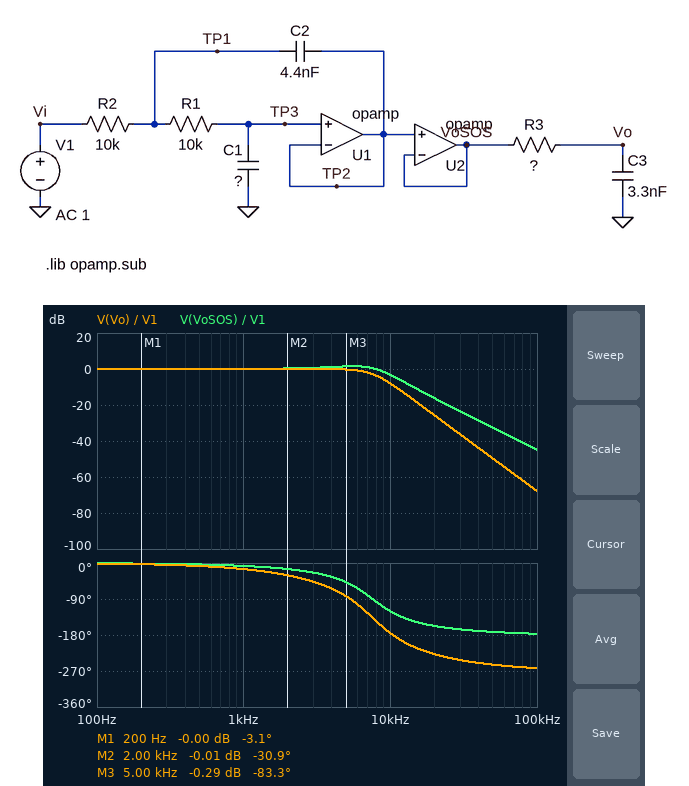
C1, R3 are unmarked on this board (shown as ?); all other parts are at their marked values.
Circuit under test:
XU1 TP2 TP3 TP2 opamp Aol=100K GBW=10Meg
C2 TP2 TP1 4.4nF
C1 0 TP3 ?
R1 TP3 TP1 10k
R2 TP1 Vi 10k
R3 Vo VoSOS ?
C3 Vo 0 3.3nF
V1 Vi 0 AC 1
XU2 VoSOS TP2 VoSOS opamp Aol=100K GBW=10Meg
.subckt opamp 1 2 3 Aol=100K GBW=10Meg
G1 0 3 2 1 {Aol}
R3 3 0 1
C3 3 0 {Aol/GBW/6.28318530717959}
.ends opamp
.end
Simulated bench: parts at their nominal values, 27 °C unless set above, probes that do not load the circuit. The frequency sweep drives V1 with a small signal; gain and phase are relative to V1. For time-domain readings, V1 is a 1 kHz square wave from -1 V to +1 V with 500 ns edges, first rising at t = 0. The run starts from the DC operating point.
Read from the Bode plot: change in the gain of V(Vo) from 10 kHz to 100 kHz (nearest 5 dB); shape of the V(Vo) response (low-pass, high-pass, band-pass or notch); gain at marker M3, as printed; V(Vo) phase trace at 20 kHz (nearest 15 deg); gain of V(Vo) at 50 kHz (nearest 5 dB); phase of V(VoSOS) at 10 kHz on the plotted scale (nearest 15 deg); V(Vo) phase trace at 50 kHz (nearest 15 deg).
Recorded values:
-60 dB
low-pass
-0.29 dB
-225 deg
-50 dB
-120 deg
-255 deg
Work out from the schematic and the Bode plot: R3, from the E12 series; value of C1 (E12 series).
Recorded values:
6.8 kΩ
1 nF
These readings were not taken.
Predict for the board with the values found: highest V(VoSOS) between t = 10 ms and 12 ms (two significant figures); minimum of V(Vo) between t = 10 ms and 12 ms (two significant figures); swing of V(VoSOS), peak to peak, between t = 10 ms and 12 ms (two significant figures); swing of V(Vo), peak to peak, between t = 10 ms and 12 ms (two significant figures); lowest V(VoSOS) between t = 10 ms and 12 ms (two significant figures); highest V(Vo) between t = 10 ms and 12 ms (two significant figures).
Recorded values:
1.4 V
-1.2 V
2.7 V
2.3 V
-1.4 V
1.2 V
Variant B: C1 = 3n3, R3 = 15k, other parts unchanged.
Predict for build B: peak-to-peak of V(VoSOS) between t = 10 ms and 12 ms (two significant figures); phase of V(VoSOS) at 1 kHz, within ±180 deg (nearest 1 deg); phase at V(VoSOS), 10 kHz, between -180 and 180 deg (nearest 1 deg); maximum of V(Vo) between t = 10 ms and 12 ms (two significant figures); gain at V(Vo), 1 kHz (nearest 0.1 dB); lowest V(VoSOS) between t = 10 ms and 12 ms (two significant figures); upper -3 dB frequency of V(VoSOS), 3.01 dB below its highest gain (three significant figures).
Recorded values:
2.0 V
-24 deg
-139 deg
1.0 V
-0.7 dB
-1.0 V
3.28 kHz
